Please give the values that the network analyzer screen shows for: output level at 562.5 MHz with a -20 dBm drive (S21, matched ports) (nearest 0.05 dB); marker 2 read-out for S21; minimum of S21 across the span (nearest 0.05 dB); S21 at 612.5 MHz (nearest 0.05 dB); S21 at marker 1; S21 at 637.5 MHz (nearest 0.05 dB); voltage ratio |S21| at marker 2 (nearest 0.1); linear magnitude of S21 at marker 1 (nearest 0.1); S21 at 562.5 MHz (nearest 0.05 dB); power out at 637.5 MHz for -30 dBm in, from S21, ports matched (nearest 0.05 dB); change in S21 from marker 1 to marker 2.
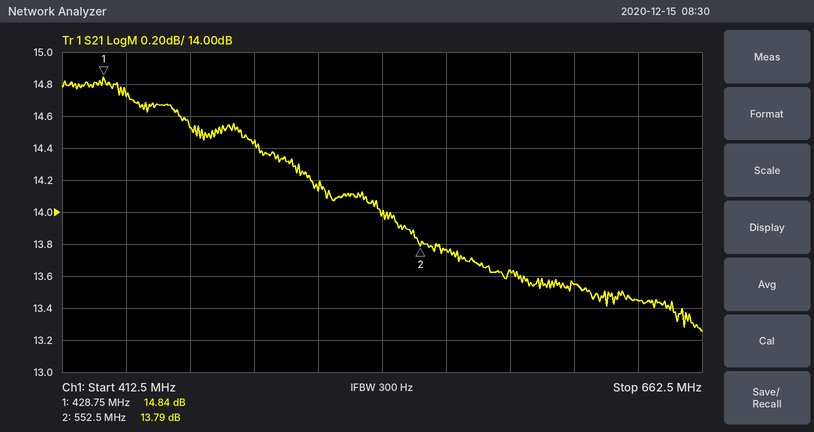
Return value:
-6.25 dBm
13.79 dB
13.25 dB
13.55 dB
14.84 dB
13.45 dB
4.9
5.5
13.75 dB
-16.55 dBm
-1.05 dB
